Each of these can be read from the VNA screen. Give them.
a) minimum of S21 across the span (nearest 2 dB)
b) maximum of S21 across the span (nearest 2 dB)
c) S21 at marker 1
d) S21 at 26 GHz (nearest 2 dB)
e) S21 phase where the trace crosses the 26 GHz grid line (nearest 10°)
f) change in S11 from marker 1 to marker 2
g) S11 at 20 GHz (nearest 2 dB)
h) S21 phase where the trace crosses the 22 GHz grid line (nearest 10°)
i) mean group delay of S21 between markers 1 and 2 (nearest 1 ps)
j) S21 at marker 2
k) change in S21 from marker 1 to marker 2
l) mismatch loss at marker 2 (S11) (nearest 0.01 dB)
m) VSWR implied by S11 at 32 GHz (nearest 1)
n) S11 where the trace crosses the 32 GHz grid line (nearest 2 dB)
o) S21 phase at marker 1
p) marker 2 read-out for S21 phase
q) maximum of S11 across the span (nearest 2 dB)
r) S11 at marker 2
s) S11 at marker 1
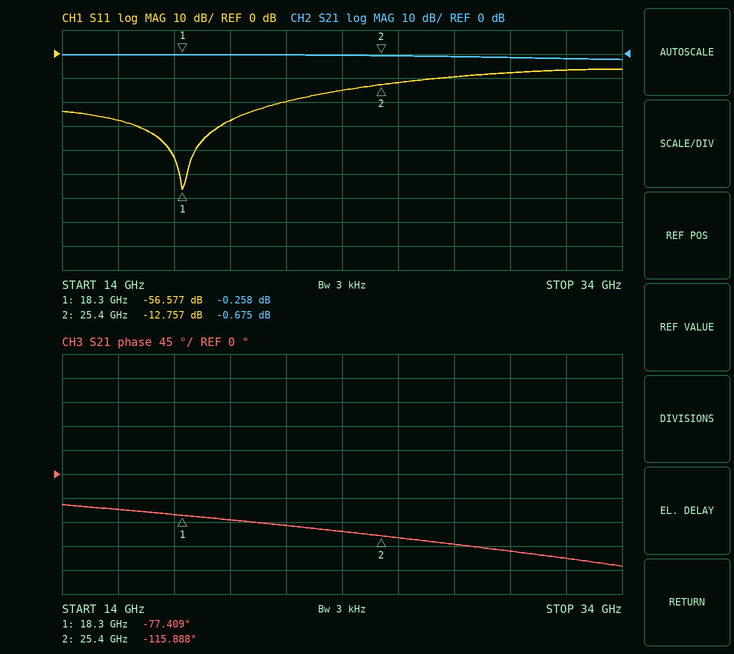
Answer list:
-2 dB
0 dB
-0.258 dB
0 dB
-120°
43.820 dB
-28 dB
-100°
15 ps
-0.675 dB
-0.417 dB
0.24 dB
3
-6 dB
-77.409°
-115.888°
-6 dB
-12.757 dB
-56.577 dB
